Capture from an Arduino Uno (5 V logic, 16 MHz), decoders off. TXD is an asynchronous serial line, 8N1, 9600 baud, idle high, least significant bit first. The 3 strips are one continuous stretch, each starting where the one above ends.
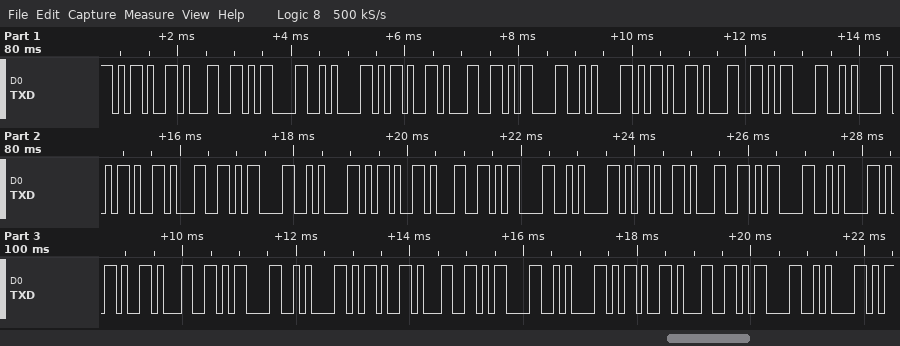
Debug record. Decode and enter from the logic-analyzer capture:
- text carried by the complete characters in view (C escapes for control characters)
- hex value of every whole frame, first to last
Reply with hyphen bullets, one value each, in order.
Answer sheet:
- "-1\r\n-1\r\n-1\r\n-1\r\n-1\r\n-1\r\n-1\r\n-1\r\n-1\r\n"
- 2D 31 0D 0A 2D 31 0D 0A 2D 31 0D 0A 2D 31 0D 0A 2D 31 0D 0A 2D 31 0D 0A 2D 31 0D 0A 2D 31 0D 0A 2D 31 0D 0A
